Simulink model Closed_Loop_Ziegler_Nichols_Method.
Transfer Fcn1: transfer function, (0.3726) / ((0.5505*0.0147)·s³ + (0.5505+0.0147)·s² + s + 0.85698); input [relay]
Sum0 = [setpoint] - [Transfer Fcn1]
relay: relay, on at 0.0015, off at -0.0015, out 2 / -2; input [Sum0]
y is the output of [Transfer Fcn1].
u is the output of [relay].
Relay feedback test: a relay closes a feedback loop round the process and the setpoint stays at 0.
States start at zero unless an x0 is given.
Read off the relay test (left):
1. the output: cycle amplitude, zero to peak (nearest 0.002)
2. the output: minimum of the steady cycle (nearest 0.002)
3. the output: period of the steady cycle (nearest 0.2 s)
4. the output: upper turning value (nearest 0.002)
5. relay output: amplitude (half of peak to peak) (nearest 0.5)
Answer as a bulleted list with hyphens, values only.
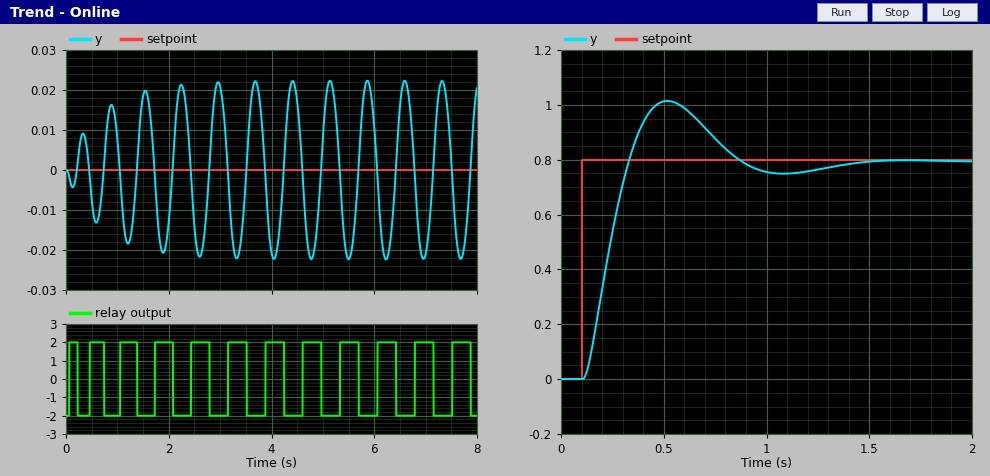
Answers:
- 0.022
- -0.022
- 0.8 s
- 0.022
- 2.0
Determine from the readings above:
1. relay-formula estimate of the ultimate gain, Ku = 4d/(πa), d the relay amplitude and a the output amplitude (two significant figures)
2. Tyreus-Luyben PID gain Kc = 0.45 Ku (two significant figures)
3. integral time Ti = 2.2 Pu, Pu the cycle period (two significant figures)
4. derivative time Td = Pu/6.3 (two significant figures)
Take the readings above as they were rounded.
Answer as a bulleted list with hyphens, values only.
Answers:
- 120
- 54
- 1.8 s
- 0.13 s
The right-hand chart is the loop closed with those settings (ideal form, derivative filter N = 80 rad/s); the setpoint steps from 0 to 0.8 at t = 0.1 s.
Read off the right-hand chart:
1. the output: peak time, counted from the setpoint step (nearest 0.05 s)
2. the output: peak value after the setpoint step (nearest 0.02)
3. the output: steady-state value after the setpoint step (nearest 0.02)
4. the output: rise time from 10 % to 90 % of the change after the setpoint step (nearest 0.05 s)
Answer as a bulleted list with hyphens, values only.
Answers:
- 0.40 s
- 1.02
- 0.80
- 0.15 s
